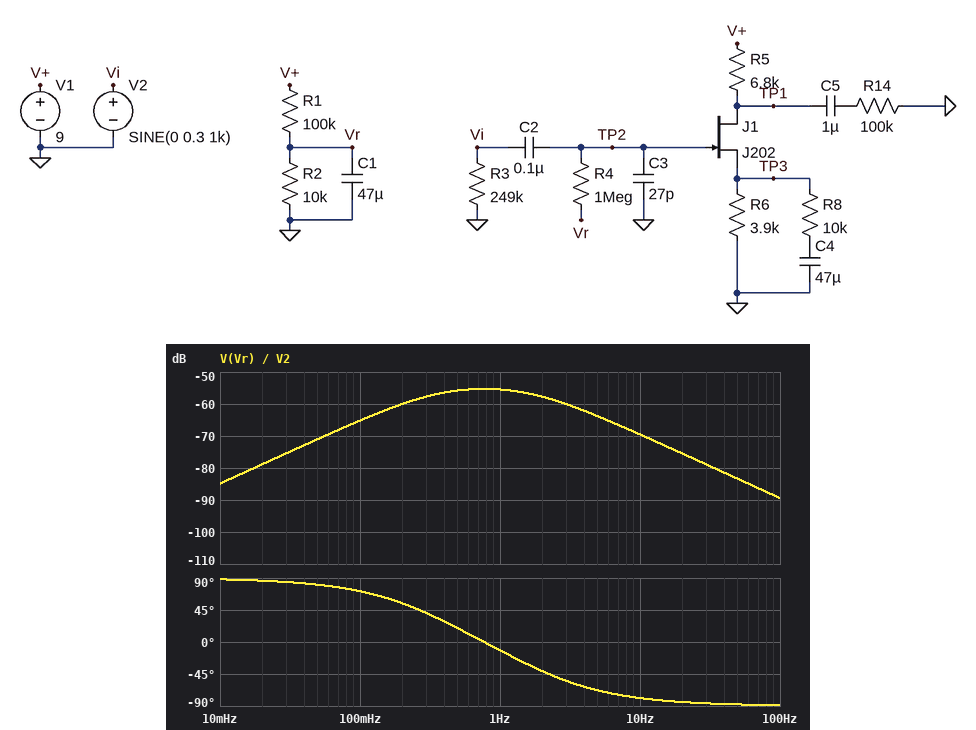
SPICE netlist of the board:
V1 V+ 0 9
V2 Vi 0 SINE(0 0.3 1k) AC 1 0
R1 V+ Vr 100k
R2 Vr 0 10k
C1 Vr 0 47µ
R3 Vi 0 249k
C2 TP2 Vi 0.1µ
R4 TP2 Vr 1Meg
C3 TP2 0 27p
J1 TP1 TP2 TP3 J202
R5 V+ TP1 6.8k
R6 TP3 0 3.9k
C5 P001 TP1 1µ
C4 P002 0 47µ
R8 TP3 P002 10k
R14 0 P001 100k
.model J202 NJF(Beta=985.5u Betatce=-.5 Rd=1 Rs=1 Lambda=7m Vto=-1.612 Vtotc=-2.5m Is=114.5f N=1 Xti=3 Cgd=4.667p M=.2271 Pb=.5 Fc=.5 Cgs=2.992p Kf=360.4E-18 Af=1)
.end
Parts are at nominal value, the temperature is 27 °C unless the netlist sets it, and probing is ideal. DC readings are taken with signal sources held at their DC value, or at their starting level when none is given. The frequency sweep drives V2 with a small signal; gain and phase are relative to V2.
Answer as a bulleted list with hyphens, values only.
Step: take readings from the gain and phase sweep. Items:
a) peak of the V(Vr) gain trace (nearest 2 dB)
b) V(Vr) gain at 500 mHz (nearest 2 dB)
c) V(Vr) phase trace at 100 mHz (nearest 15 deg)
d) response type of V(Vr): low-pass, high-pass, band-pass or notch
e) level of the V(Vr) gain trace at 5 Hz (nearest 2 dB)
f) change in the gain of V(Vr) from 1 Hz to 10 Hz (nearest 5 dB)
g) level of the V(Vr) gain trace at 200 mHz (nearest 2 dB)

- -56 dB
- -56 dB
- 75 deg
- band-pass
- -64 dB
- -15 dB
- -60 dB
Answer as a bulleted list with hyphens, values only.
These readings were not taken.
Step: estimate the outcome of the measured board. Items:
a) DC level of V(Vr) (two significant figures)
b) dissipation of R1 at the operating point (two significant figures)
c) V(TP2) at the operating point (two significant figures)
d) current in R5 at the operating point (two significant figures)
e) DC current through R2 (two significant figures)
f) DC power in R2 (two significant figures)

- 820 mV
- 670 µW
- 820 mV
- 450 µA
- 82 µA
- 67 µW
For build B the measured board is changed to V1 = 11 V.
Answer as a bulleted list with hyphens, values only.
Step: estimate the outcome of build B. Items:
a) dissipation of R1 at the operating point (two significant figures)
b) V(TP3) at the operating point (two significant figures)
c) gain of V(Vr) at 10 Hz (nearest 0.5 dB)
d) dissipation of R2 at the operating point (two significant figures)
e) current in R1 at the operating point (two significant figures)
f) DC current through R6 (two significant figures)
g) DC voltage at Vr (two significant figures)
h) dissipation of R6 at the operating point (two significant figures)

- 1.0 mW
- 1.9 V
- -69.5 dB
- 100 µW
- 100 µA
- 490 µA
- 1.0 V
- 940 µW
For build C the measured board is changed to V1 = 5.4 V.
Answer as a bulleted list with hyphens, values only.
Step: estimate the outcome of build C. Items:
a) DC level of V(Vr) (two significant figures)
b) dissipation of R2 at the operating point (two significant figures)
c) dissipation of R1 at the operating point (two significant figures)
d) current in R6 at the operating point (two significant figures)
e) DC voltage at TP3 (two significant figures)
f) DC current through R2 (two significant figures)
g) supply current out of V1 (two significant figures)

- 490 mV
- 24 µW
- 240 µW
- 380 µA
- 1.5 V
- 49 µA
- 430 µA
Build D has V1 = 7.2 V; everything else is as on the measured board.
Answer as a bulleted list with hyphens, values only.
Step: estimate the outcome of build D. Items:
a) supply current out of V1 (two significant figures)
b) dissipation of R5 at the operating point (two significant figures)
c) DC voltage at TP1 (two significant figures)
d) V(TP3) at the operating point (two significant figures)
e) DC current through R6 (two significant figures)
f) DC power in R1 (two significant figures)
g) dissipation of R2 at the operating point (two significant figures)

- 480 µA
- 1.2 mW
- 4.4 V
- 1.6 V
- 420 µA
- 430 µW
- 43 µW
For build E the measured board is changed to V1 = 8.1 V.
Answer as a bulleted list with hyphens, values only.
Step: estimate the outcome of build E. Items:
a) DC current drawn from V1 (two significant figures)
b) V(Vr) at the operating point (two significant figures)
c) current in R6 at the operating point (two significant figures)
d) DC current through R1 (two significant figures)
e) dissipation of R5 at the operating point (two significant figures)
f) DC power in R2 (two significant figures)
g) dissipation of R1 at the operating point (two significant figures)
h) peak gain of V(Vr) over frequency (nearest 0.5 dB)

- 510 µA
- 740 mV
- 430 µA
- 74 µA
- 1.3 mW
- 54 µW
- 540 µW
- -55.5 dB
